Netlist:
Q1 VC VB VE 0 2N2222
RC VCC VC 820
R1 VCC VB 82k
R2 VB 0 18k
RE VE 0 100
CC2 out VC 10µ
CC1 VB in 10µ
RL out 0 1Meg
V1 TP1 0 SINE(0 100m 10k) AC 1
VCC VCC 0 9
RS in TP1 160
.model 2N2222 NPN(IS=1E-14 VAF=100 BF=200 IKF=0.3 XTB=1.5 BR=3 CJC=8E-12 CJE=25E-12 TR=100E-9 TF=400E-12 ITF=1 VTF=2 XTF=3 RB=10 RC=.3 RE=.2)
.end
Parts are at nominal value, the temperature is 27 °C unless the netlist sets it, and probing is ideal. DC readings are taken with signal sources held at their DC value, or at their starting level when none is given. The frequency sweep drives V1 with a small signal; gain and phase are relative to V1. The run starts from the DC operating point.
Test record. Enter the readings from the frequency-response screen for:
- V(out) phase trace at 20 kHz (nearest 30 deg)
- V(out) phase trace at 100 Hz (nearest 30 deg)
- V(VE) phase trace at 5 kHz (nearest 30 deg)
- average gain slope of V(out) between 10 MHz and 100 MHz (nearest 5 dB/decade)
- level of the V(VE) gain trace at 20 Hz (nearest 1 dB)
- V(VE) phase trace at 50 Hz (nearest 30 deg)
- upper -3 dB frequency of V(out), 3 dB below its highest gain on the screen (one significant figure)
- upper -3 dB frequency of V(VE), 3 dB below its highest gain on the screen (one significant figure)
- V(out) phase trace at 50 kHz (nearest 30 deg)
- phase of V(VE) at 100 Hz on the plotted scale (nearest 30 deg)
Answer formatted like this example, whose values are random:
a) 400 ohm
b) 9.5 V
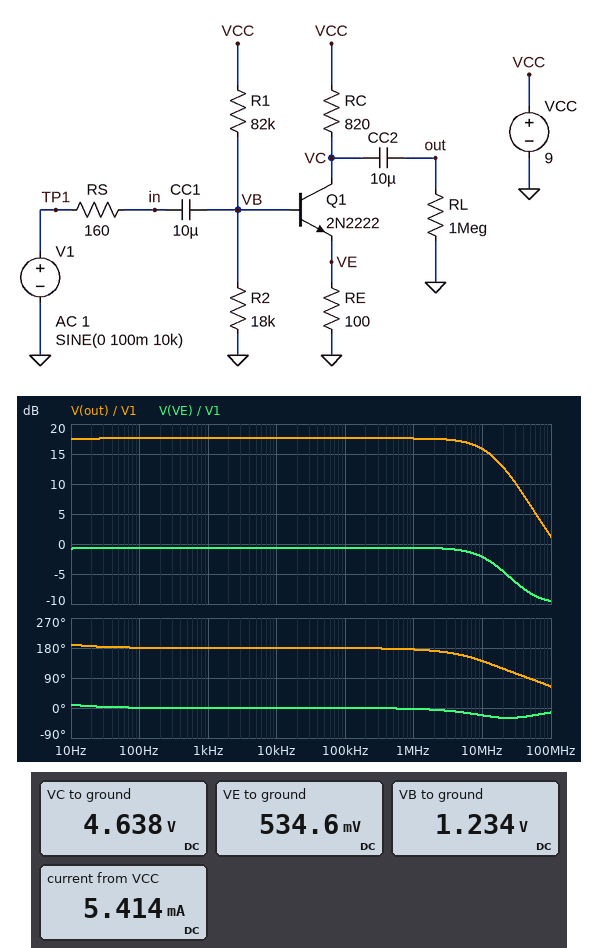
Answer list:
a) 180 deg
b) 180 deg
c) 0 deg
d) -15 dB/decade
e) -1 dB
f) 0 deg
g) 10 MHz
h) 20 MHz
i) 180 deg
j) 0 deg
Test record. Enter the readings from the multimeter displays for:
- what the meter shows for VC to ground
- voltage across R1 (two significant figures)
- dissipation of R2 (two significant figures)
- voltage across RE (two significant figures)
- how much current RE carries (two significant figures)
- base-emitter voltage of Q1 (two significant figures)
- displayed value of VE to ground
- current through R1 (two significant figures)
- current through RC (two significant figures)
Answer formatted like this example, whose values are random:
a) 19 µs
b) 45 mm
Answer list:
a) 4.638 V
b) 7.8 V
c) 85 µW
d) 530 mV
e) 5.3 mA
f) 700 mV
g) 534.6 mV
h) 95 µA
i) 5.3 mA
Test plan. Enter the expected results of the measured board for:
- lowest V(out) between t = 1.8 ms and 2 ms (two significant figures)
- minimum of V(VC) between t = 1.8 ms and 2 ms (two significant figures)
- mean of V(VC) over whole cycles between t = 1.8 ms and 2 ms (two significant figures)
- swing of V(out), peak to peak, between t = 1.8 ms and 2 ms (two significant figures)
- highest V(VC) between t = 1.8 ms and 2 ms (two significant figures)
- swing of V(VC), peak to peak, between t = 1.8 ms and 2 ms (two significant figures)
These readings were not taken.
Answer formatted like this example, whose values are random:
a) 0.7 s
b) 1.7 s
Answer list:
a) -760 mV
b) 3.9 V
c) 4.6 V
d) 1.5 V
e) 5.4 V
f) 1.5 V
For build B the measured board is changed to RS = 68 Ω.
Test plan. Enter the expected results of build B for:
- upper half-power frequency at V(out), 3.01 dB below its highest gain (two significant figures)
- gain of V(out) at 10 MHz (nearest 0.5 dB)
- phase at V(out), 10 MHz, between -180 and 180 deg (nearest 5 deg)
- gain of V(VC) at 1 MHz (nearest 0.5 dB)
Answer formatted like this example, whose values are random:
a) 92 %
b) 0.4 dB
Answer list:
a) 22 MHz
b) 17.0 dB
c) 150 deg
d) 17.5 dB
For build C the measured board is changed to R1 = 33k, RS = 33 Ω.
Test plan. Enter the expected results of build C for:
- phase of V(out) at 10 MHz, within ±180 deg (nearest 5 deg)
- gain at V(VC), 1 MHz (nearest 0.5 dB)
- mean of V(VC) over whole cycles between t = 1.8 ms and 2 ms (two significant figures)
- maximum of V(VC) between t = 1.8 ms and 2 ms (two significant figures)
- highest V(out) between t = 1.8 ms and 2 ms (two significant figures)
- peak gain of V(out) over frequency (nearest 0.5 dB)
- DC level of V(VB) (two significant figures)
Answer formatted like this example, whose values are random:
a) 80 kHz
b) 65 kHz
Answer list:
a) 10 deg
b) -1.5 dB
c) 1.4 V
d) 2.0 V
e) 880 mV
f) 1.0 dB
g) 1.7 V
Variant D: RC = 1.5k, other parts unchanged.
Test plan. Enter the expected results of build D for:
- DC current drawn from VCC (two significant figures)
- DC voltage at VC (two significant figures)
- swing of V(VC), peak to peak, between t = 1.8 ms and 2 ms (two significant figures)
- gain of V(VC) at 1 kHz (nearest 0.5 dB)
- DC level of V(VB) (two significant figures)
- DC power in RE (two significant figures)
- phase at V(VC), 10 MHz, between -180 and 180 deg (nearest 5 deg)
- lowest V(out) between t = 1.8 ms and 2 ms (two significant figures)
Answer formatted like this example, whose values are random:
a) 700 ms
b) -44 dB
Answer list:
a) 5.3 mA
b) 1.1 V
c) 2.0 V
d) 23.0 dB
e) 1.2 V
f) 2.8 mW
g) 110 deg
h) -500 mV
